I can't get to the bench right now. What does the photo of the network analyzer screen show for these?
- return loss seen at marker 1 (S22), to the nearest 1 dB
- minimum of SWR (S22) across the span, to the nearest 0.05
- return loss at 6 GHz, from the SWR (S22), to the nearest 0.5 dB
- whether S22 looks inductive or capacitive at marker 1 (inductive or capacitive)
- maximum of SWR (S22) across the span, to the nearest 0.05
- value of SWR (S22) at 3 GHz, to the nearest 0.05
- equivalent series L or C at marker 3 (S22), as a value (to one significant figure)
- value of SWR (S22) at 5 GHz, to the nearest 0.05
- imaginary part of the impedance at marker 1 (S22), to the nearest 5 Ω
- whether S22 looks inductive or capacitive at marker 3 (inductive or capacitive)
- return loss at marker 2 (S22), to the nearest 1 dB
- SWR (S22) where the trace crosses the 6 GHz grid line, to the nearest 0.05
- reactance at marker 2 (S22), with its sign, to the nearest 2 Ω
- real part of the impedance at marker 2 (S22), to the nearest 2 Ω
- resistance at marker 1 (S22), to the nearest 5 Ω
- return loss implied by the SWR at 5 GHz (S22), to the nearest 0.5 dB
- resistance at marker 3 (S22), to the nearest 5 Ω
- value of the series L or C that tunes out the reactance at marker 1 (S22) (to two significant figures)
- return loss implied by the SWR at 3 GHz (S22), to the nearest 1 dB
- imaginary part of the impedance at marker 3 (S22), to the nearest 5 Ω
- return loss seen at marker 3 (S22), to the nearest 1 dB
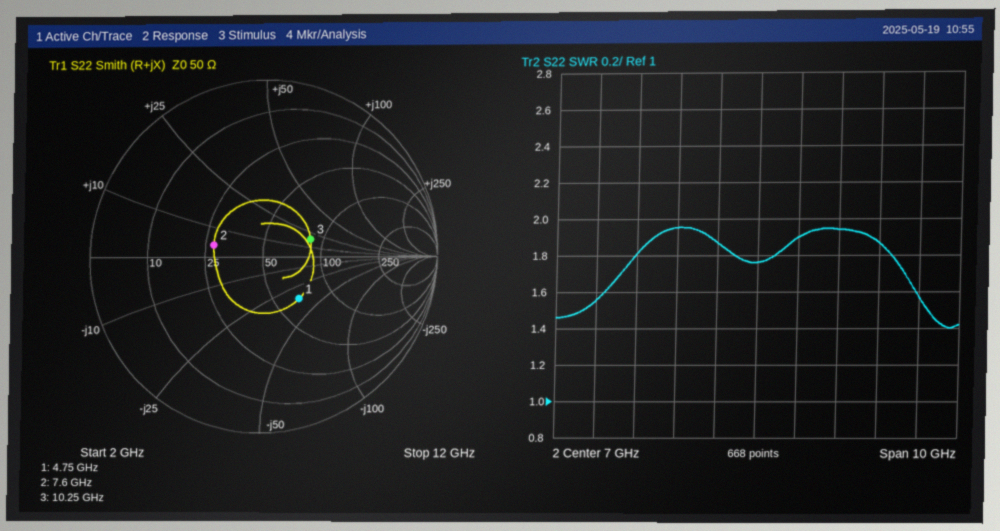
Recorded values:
10 dB
1.40
10.5 dB
capacitive
1.95
1.55
300 pH
1.95
-35 Ω
inductive
11 dB
1.85
+4 Ω
28 Ω
65 Ω
10.0 dB
85 Ω
1.2 nH
13 dB
+20 Ω
11 dB
